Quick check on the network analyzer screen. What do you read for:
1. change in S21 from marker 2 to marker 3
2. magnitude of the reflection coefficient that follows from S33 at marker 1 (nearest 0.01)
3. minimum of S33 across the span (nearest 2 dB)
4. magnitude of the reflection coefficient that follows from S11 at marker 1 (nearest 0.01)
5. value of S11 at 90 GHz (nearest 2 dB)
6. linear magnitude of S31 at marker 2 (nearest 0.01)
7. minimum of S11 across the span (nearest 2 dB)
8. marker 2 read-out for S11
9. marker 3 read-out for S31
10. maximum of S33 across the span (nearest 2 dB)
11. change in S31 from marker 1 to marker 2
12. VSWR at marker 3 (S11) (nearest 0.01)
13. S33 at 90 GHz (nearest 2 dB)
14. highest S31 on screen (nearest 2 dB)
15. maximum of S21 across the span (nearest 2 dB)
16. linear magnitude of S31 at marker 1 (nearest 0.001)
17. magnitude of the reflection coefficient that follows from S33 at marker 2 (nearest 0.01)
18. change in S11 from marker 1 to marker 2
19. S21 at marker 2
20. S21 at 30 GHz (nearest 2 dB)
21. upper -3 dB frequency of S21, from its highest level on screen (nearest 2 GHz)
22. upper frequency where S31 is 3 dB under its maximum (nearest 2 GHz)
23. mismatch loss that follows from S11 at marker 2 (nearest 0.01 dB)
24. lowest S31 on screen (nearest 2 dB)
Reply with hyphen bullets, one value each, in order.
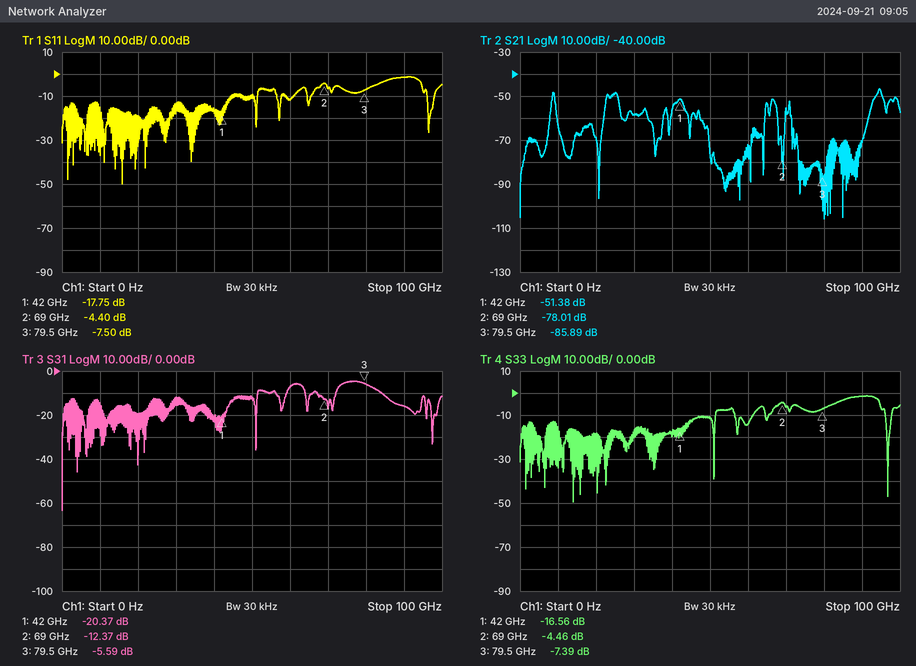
- -7.88 dB
- 0.15
- -50 dB
- 0.13
- -2 dB
- 0.24
- -50 dB
- -4.40 dB
- -5.59 dB
- -2 dB
- 8.00 dB
- 2.46
- -2 dB
- -4 dB
- -46 dB
- 0.096
- 0.60
- 13.35 dB
- -78.01 dB
- -58 dB
- 96 GHz
- 82 GHz
- 1.96 dB
- -64 dB
